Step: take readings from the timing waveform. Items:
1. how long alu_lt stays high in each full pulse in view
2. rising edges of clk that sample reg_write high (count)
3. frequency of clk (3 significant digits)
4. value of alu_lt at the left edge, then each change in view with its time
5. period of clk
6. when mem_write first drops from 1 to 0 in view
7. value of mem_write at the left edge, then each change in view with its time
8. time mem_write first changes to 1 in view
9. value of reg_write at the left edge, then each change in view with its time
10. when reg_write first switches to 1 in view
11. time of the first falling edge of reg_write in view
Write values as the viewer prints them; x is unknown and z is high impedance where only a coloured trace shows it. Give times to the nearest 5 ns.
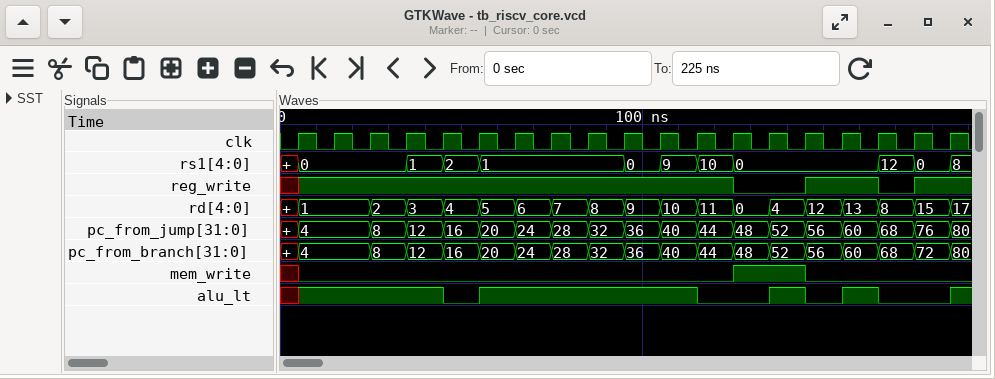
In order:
60 ns, 10 ns, 10 ns
15
100 MHz
x, 1 at 5 ns, 0 at 45 ns, 1 at 55 ns, 0 at 115 ns, 1 at 135 ns, 0 at 145 ns, 1 at 155 ns, 0 at 165 ns, 1 at 185 ns
10 ns
145 ns
x, 0 at 5 ns, 1 at 125 ns, 0 at 145 ns
125 ns
x, 1 at 5 ns, 0 at 125 ns, 1 at 145 ns, 0 at 165 ns, 1 at 175 ns
5 ns
125 ns
